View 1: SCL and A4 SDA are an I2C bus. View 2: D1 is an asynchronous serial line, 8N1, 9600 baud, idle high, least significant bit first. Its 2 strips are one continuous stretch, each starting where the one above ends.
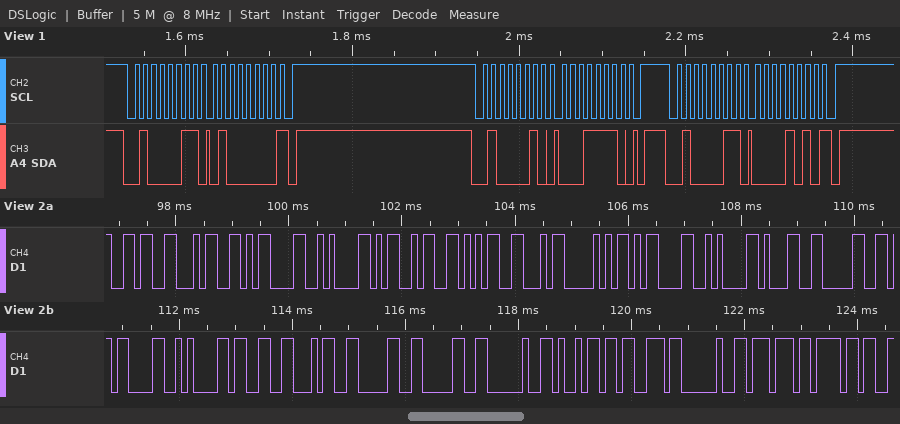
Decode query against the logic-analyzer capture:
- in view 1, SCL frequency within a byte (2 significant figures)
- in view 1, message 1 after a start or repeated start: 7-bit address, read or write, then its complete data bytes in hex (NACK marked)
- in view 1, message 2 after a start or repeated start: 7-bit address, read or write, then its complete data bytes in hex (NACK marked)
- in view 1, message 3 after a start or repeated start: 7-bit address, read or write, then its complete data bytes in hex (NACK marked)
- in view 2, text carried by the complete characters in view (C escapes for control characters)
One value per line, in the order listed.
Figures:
100 kHz
0x21 read: 40 NACK
0x21 write: 1E
0x21 read: 0A NACK
"64\r\nMVFP\r\n10\r\n3400 is wo"
